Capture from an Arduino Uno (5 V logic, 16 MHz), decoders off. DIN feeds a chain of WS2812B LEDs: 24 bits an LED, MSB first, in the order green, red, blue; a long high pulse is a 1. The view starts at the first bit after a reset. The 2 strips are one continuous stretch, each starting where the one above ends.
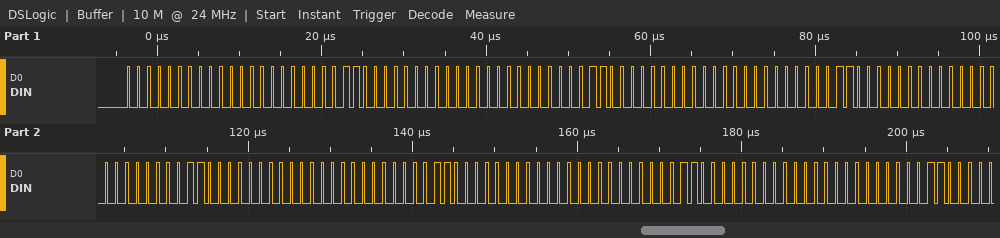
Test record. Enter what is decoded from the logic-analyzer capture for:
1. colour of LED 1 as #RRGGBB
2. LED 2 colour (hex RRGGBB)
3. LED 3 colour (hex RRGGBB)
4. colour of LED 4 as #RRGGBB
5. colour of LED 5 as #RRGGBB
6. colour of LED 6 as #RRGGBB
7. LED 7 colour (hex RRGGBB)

#000006
#000006
#000006
#000006
#000006
#000006
#000006
